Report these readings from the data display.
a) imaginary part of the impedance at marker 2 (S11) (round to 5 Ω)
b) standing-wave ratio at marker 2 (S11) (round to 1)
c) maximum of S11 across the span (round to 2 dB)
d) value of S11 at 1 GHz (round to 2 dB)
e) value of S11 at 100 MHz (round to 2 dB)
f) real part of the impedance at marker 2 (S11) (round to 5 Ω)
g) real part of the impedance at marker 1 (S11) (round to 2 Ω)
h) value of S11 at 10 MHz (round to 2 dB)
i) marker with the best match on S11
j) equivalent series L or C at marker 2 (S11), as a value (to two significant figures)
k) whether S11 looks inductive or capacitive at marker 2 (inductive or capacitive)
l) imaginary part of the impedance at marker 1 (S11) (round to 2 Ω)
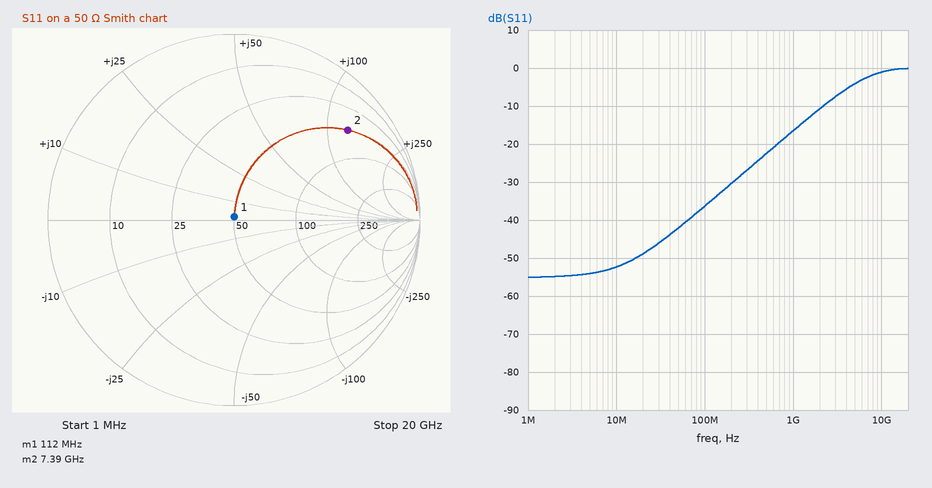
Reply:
+125 Ω
8
0 dB
-16 dB
-36 dB
50 Ω
50 Ω
-52 dB
marker 1
2.7 nH
inductive
+2 Ω
